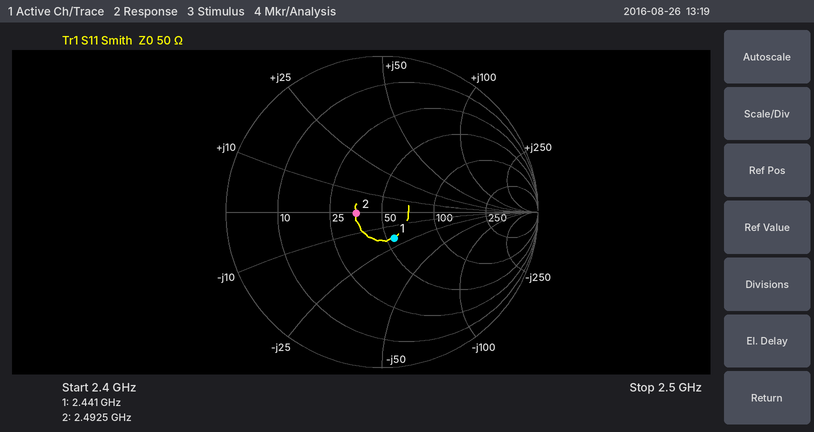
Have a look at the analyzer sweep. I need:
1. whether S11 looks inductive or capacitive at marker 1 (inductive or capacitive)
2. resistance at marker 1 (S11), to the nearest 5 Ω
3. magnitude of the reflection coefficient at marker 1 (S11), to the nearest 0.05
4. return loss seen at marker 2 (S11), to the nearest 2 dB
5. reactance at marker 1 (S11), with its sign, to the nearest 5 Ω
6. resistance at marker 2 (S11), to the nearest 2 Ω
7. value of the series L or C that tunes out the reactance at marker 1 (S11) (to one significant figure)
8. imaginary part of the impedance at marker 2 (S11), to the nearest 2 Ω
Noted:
capacitive
55 Ω
0.20
16 dB
-20 Ω
36 Ω
1 nH
0 Ω
